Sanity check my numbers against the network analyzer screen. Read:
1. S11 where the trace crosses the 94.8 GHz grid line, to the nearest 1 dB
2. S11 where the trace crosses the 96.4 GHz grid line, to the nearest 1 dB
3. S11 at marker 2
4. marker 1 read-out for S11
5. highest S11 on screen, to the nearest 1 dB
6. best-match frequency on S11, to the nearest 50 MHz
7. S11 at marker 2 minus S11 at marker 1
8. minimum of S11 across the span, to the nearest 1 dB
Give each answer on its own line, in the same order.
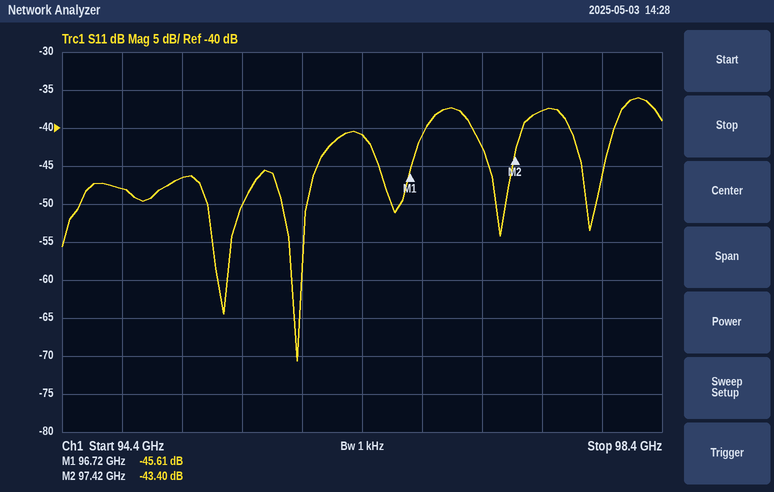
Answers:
-48 dB
-41 dB
-43.40 dB
-45.61 dB
-36 dB
95.95 GHz
2.21 dB
-71 dB
